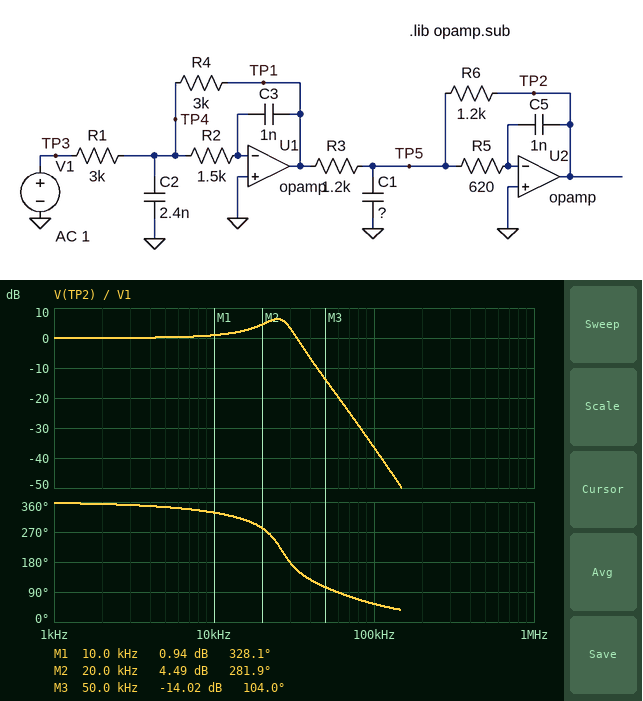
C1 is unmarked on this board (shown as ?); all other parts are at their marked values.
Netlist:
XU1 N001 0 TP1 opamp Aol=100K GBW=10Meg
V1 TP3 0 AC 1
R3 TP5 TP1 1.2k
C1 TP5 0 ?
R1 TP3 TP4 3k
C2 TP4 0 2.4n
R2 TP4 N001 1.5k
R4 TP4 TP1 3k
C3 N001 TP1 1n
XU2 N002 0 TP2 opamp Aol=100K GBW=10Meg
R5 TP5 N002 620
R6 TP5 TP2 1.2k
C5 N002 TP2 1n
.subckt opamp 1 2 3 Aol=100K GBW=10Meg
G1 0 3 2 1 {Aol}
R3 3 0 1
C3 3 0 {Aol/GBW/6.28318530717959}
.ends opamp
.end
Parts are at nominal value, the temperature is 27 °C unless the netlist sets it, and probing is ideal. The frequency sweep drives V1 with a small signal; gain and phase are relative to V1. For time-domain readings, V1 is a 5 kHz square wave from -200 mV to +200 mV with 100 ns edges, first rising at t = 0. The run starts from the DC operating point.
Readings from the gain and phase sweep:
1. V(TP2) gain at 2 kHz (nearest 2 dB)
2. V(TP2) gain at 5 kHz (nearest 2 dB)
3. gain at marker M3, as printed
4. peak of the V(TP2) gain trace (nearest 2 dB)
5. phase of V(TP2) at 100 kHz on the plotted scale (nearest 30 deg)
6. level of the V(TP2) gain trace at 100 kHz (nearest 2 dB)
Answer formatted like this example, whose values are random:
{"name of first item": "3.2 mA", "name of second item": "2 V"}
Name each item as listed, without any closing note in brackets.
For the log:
{"V(TP2) gain at 2 kHz": "0 dB", "V(TP2) gain at 5 kHz": "0 dB", "gain at marker M3, as printed": "-14.02 dB", "peak of the V(TP2) gain trace": "6 dB", "phase of V(TP2) at 100 kHz on the plotted scale": "60 deg", "level of the V(TP2) gain trace at 100 kHz": "-36 dB"}
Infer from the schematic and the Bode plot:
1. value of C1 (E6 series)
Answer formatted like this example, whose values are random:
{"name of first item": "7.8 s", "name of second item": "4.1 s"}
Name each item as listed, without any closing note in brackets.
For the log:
{"value of C1": "47 nF"}
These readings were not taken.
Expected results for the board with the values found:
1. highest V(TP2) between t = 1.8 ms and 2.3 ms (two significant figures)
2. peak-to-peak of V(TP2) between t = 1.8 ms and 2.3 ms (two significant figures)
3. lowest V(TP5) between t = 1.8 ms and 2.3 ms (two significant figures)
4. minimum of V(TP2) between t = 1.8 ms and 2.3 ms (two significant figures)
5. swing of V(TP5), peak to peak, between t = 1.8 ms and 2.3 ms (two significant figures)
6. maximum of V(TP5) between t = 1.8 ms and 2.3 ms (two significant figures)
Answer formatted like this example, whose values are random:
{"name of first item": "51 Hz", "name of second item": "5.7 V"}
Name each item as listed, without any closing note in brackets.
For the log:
{"highest V(TP2) between t = 1.8 ms and 2.3 ms": "370 mV", "peak-to-peak of V(TP2) between t = 1.8 ms and 2.3 ms": "740 mV", "lowest V(TP5) between t = 1.8 ms and 2.3 ms": "-27 mV", "minimum of V(TP2) between t = 1.8 ms and 2.3 ms": "-370 mV", "swing of V(TP5), peak to peak, between t = 1.8 ms and 2.3 ms": "54 mV", "maximum of V(TP5) between t = 1.8 ms and 2.3 ms": "27 mV"}
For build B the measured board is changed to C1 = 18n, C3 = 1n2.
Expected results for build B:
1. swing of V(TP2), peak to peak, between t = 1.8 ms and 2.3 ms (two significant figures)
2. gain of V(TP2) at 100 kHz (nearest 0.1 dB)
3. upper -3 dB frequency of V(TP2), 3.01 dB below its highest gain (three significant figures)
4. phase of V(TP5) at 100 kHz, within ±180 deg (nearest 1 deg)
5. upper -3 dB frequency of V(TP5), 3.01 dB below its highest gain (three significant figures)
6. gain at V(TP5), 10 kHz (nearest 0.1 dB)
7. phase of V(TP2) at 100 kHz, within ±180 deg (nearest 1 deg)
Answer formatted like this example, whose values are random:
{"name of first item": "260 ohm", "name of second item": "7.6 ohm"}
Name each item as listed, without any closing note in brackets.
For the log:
{"swing of V(TP2), peak to peak, between t = 1.8 ms and 2.3 ms": "490 mV", "gain of V(TP2) at 100 kHz": "-29.2 dB", "upper -3 dB frequency of V(TP2), 3.01 dB below its highest gain": "44.8 kHz", "phase of V(TP5) at 100 kHz, within ±180 deg": "-24 deg", "upper -3 dB frequency of V(TP5), 3.01 dB below its highest gain": "50.9 kHz", "gain at V(TP5), 10 kHz": "-28.0 dB", "phase of V(TP2) at 100 kHz, within ±180 deg": "66 deg"}
